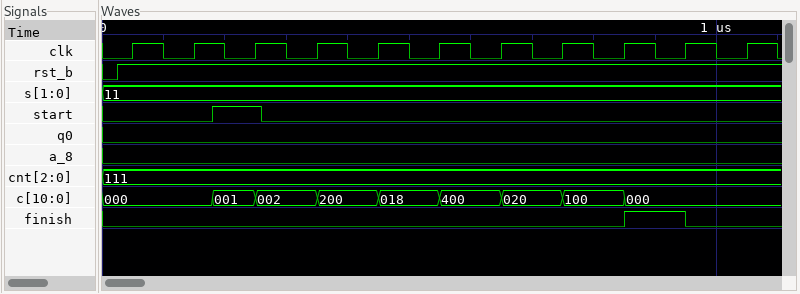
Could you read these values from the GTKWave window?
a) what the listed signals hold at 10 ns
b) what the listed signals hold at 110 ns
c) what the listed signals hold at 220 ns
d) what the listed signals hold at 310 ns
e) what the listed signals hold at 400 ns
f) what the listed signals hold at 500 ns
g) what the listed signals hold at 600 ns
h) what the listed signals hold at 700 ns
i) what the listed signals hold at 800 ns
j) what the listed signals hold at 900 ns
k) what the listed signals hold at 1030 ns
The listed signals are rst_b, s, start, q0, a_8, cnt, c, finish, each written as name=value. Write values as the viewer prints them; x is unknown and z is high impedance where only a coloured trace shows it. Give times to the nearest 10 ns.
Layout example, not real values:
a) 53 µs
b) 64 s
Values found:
a) rst_b=0, s=11, start=0, q0=0, a_8=0, cnt=111, c=000, finish=0
b) rst_b=1, s=11, start=0, q0=0, a_8=0, cnt=111, c=000, finish=0
c) rst_b=1, s=11, start=1, q0=0, a_8=0, cnt=111, c=001, finish=0
d) rst_b=1, s=11, start=0, q0=0, a_8=0, cnt=111, c=002, finish=0
e) rst_b=1, s=11, start=0, q0=0, a_8=0, cnt=111, c=200, finish=0
f) rst_b=1, s=11, start=0, q0=0, a_8=0, cnt=111, c=018, finish=0
g) rst_b=1, s=11, start=0, q0=0, a_8=0, cnt=111, c=400, finish=0
h) rst_b=1, s=11, start=0, q0=0, a_8=0, cnt=111, c=020, finish=0
i) rst_b=1, s=11, start=0, q0=0, a_8=0, cnt=111, c=100, finish=0
j) rst_b=1, s=11, start=0, q0=0, a_8=0, cnt=111, c=000, finish=1
k) rst_b=1, s=11, start=0, q0=0, a_8=0, cnt=111, c=000, finish=0
